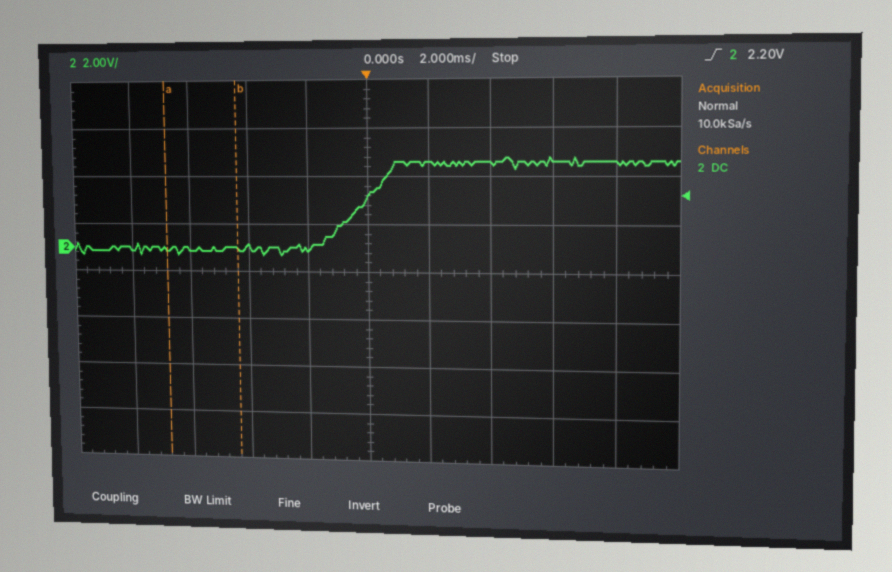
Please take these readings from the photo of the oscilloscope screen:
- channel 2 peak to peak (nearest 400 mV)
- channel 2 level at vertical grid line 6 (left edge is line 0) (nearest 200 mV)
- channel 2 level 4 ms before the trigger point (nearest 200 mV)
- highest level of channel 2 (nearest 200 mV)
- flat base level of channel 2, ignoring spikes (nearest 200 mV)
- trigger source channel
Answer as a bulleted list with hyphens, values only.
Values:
- 4.0 V
- 3.6 V
- 0.0 V
- 3.8 V
- 0.0 V
- channel 2
